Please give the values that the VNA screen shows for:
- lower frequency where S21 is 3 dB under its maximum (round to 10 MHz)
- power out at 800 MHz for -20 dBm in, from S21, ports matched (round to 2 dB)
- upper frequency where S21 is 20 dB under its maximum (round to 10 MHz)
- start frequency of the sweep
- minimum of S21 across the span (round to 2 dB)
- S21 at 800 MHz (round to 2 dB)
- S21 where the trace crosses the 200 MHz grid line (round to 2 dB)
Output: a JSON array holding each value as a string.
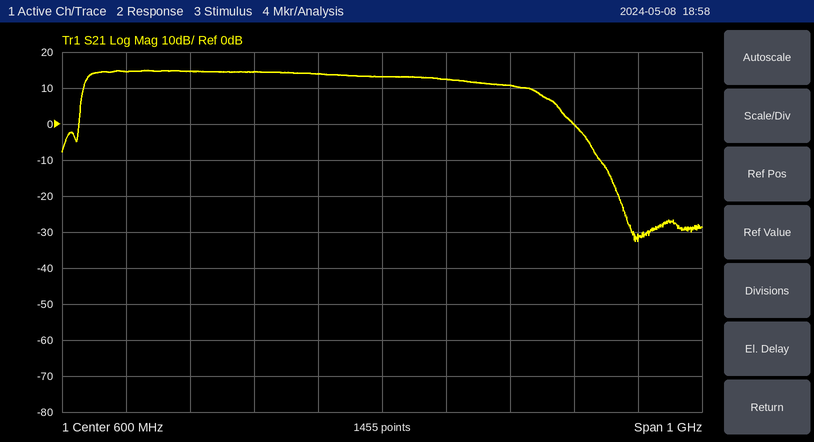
["140 MHz", "-10 dBm", "920 MHz", "100 MHz", "-32 dB", "10 dB", "14 dB"]
